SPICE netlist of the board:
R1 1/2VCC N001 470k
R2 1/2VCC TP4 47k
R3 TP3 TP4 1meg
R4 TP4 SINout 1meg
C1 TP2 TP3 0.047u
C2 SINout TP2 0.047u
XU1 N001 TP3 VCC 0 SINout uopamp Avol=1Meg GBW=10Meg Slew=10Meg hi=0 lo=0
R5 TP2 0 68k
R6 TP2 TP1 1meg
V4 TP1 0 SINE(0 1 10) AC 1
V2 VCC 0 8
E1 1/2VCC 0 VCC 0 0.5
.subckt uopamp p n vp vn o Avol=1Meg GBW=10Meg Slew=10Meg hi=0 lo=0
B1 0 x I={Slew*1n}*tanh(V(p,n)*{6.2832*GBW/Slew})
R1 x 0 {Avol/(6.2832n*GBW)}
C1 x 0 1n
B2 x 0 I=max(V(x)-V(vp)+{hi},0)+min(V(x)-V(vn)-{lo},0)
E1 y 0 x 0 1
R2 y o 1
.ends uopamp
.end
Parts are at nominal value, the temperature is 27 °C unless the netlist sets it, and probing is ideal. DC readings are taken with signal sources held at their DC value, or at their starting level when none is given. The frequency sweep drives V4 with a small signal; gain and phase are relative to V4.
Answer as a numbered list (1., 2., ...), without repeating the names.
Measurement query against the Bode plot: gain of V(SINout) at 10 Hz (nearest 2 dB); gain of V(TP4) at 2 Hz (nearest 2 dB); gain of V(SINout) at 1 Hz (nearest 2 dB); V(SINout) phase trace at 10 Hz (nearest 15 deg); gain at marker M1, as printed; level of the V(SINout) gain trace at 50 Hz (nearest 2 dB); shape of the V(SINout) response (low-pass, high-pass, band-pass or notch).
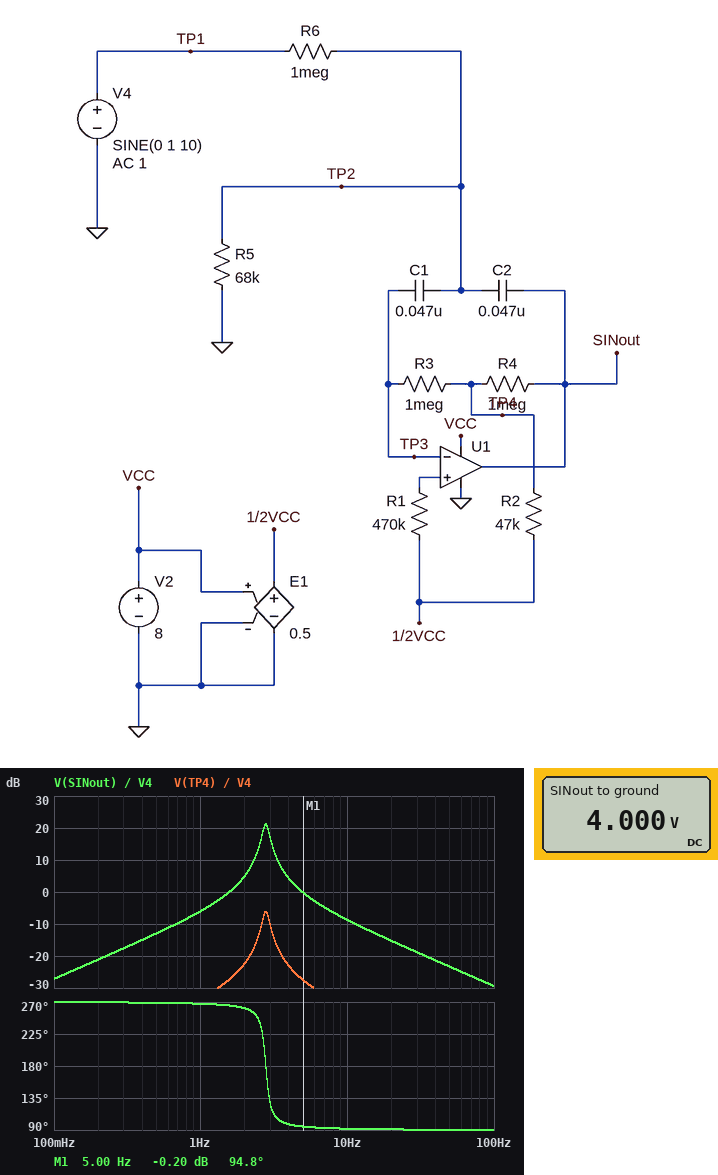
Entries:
1. -8 dB
2. -22 dB
3. -6 dB
4. 90 deg
5. -0.20 dB
6. -24 dB
7. band-pass
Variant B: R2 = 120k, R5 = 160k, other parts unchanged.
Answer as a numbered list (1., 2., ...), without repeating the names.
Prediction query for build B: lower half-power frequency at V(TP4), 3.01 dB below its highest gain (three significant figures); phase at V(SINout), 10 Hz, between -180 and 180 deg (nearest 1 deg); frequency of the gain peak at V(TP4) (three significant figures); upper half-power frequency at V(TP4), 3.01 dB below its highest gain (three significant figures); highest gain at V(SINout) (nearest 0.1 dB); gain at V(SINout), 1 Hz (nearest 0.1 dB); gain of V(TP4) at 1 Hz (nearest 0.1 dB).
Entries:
1. 2.53 Hz
2. 94 deg
3. 2.84 Hz
4. 3.18 Hz
5. 14.3 dB
6. -6.4 dB
7. -26.7 dB
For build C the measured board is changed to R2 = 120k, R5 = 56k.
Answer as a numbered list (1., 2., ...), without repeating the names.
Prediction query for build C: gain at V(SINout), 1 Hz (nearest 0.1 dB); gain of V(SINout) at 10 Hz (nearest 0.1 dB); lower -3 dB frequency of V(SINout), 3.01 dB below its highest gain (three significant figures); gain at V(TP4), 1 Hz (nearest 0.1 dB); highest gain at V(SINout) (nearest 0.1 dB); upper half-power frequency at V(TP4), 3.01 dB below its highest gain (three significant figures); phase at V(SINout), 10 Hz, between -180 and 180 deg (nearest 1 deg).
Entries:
1. -15.4 dB
2. -7.4 dB
3. 4.26 Hz
4. -35.7 dB
5. 14.3 dB
6. 4.91 Hz
7. 95 deg
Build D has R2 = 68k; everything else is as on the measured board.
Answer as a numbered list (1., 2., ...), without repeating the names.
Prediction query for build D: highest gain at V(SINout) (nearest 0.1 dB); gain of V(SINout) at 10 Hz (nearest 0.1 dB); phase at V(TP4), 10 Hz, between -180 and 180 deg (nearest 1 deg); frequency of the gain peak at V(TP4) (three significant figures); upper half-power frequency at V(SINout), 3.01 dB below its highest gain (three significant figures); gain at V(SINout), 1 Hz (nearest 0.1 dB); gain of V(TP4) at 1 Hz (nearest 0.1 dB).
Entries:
1. 18.4 dB
2. -8.4 dB
3. 93 deg
4. 3.28 Hz
5. 3.49 Hz
6. -9.2 dB
7. -33.7 dB
